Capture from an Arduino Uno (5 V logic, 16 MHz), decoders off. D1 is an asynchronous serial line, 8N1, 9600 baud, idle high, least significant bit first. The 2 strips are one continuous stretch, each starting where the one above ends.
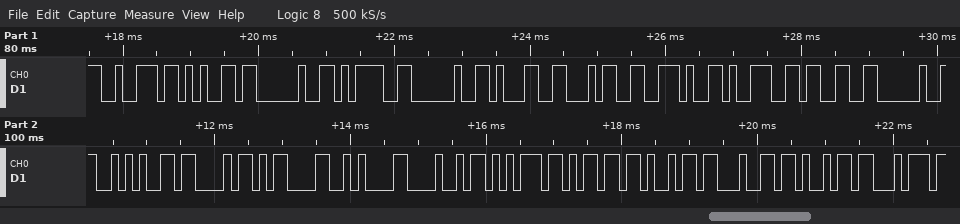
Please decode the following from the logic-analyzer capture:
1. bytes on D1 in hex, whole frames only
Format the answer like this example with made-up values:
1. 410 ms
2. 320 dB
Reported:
1. 72 65 20 3D 20 31 34 2E 39 33 20 2A 43 0D 0A 48 75 6D 69 64 69 74
